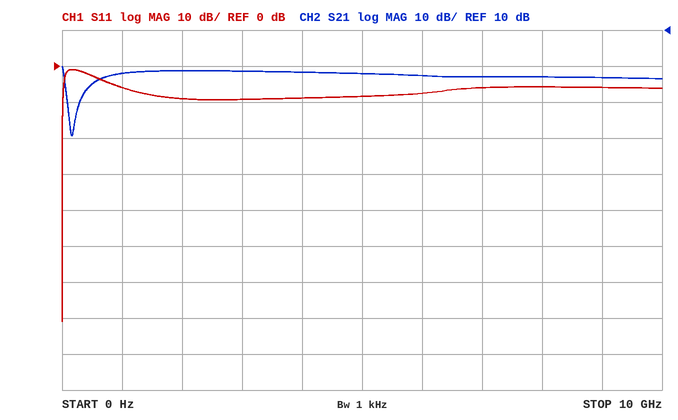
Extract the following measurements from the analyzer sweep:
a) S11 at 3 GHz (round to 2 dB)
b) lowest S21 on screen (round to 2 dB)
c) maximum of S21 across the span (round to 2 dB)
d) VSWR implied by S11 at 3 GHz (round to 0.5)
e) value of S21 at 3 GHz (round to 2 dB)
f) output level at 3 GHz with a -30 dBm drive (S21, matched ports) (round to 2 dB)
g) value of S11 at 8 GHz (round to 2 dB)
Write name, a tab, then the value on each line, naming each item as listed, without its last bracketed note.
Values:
S11 at 3 GHz	-10 dB
lowest S21 on screen	-20 dB
maximum of S21 across the span	0 dB
VSWR implied by S11 at 3 GHz	2.0
value of S21 at 3 GHz	-2 dB
output level at 3 GHz with a -30 dBm drive (S21, matched ports)	-32 dBm
value of S11 at 8 GHz	-6 dB
